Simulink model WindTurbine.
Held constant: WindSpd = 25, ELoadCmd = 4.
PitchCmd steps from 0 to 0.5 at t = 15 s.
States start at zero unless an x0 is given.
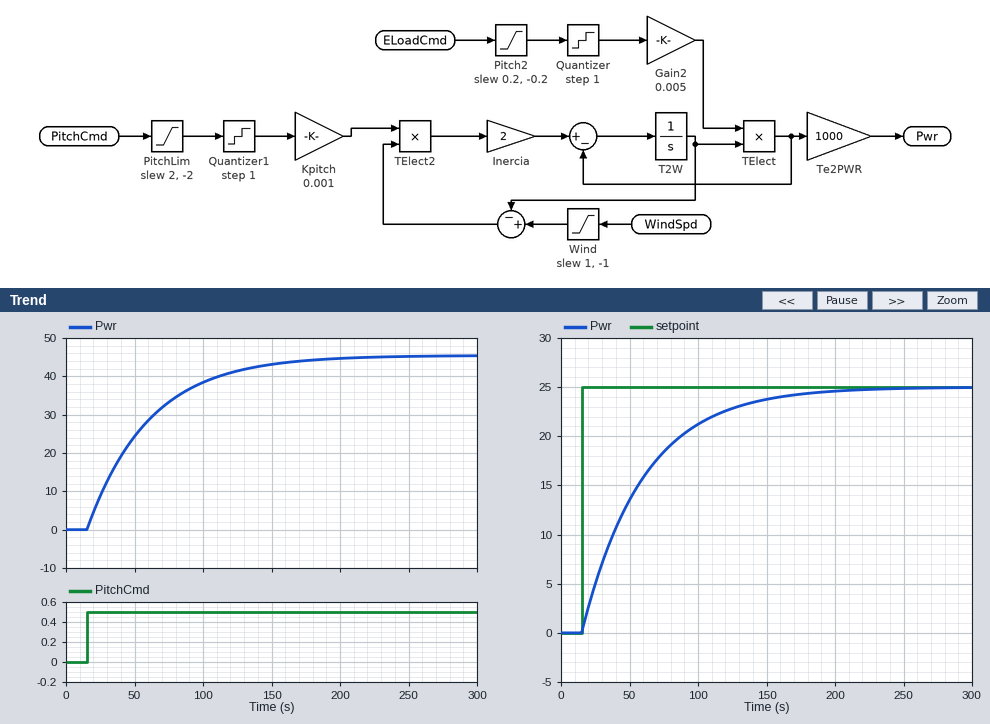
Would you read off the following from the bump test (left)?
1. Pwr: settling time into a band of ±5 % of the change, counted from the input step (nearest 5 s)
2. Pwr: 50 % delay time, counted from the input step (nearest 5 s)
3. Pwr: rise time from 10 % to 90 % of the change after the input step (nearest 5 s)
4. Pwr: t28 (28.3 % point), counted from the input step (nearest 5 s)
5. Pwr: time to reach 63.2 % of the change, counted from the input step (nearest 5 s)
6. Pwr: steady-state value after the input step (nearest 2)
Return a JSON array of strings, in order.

["135 s", "30 s", "100 s", "15 s", "45 s", "46"]
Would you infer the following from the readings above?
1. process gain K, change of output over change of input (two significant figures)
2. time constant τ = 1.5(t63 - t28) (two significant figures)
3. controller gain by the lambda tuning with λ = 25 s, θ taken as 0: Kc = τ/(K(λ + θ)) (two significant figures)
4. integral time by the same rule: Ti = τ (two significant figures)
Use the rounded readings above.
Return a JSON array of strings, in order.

["92", "45 s", "0.020", "45 s"]
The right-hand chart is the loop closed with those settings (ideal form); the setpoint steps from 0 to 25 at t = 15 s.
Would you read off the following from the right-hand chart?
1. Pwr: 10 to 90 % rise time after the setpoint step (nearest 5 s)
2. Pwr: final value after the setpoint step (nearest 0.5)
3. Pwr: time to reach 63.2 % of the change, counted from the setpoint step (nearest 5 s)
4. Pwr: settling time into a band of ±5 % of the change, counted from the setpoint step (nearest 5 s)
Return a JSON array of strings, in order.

["100 s", "25.0", "45 s", "135 s"]
